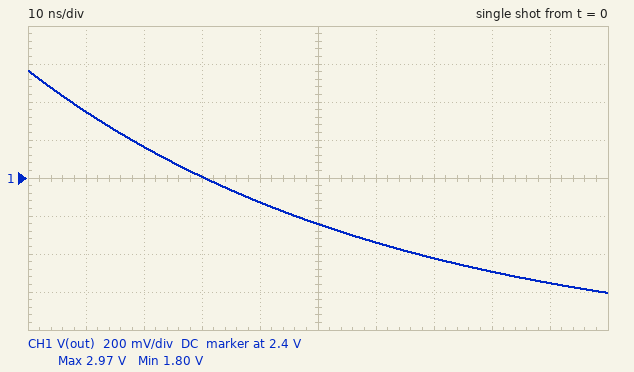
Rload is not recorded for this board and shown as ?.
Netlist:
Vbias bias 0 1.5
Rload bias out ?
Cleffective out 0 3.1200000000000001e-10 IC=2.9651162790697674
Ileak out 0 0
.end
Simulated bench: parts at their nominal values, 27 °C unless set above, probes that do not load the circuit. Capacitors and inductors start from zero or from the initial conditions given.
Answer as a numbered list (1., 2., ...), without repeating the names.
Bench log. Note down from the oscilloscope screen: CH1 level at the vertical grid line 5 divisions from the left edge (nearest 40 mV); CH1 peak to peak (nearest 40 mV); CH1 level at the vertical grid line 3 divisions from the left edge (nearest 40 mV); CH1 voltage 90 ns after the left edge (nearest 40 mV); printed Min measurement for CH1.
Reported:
1. 2.16 V
2. 1.16 V
3. 2.40 V
4. 1.84 V
5. 1.80 V
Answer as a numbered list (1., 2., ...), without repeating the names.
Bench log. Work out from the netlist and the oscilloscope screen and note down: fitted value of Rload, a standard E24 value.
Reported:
1. 200 Ω
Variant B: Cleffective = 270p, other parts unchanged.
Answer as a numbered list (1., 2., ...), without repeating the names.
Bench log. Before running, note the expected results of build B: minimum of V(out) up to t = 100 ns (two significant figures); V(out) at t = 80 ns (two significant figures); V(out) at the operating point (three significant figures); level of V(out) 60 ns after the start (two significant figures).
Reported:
1. 1.7 V
2. 1.8 V
3. 1.50 V
4. 2.0 V
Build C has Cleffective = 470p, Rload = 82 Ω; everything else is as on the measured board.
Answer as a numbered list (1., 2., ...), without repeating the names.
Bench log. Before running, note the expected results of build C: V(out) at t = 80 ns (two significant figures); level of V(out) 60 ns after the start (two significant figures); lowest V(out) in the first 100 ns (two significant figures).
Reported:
1. 1.7 V
2. 1.8 V
3. 1.6 V
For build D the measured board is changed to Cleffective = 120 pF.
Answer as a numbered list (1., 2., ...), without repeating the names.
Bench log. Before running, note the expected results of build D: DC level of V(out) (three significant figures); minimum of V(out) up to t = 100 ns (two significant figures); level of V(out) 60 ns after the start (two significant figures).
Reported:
1. 1.50 V
2. 1.5 V
3. 1.6 V
